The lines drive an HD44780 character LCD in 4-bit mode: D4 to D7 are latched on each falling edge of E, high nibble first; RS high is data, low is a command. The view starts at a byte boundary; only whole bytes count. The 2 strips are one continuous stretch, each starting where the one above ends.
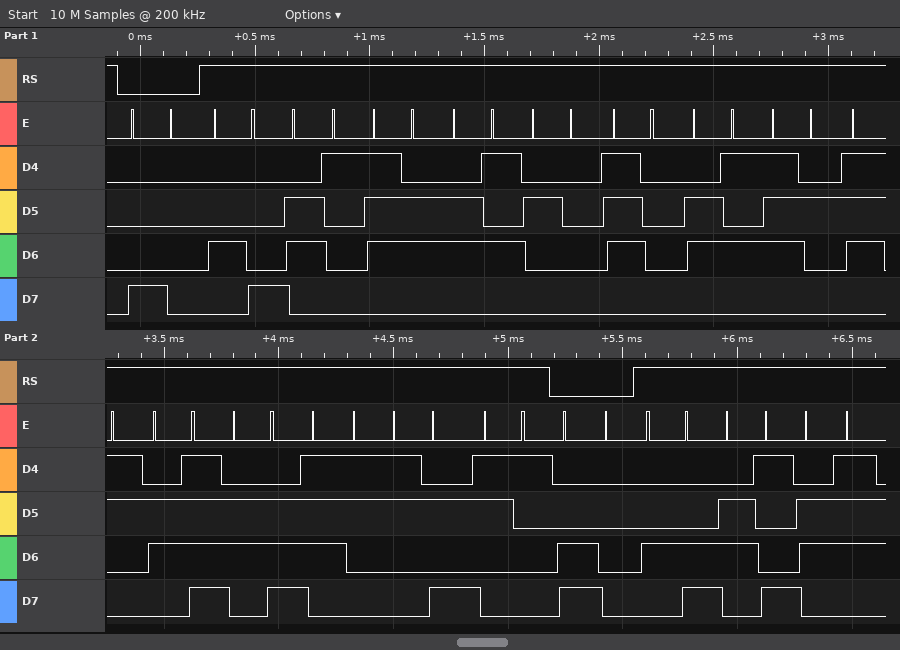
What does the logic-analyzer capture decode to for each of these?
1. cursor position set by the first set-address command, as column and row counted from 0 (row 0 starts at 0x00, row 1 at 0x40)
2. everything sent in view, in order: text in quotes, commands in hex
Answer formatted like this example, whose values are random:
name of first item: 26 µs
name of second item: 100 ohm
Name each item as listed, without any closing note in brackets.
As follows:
cursor position set by the first set-address command, as column and row counted from 0: column 0, row 0
everything sent in view, in order: text in quotes, commands in hex: 0x80 "Have persons:1" 0xC0 "Lig"
